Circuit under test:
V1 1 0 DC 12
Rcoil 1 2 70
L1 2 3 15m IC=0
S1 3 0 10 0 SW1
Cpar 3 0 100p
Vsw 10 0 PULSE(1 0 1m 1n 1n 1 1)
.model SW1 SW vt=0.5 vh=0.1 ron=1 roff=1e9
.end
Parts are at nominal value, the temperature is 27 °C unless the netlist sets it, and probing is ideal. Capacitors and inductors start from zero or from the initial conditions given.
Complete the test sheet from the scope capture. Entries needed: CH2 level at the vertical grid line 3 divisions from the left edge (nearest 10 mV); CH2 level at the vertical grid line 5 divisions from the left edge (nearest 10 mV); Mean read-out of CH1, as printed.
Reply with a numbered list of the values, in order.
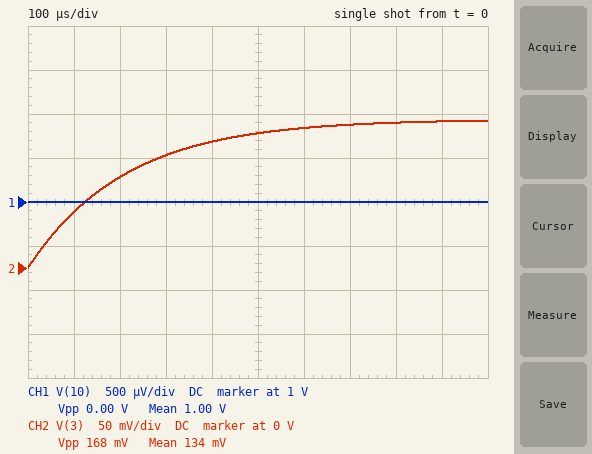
1. 130 mV
2. 150 mV
3. 1.00 V
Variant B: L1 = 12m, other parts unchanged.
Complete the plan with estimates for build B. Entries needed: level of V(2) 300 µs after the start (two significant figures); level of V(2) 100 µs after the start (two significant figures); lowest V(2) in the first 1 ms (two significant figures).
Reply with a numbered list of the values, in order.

1. 2.2 V
2. 6.7 V
3. 200 mV
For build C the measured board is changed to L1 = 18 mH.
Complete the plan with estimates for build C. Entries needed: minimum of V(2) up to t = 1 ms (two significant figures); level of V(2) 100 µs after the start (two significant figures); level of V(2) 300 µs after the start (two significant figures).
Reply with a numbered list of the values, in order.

1. 400 mV
2. 8.1 V
3. 3.8 V
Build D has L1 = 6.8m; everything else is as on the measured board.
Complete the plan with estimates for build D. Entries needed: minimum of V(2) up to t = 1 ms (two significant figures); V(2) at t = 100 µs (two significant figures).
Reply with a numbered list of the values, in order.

1. 170 mV
2. 4.3 V
